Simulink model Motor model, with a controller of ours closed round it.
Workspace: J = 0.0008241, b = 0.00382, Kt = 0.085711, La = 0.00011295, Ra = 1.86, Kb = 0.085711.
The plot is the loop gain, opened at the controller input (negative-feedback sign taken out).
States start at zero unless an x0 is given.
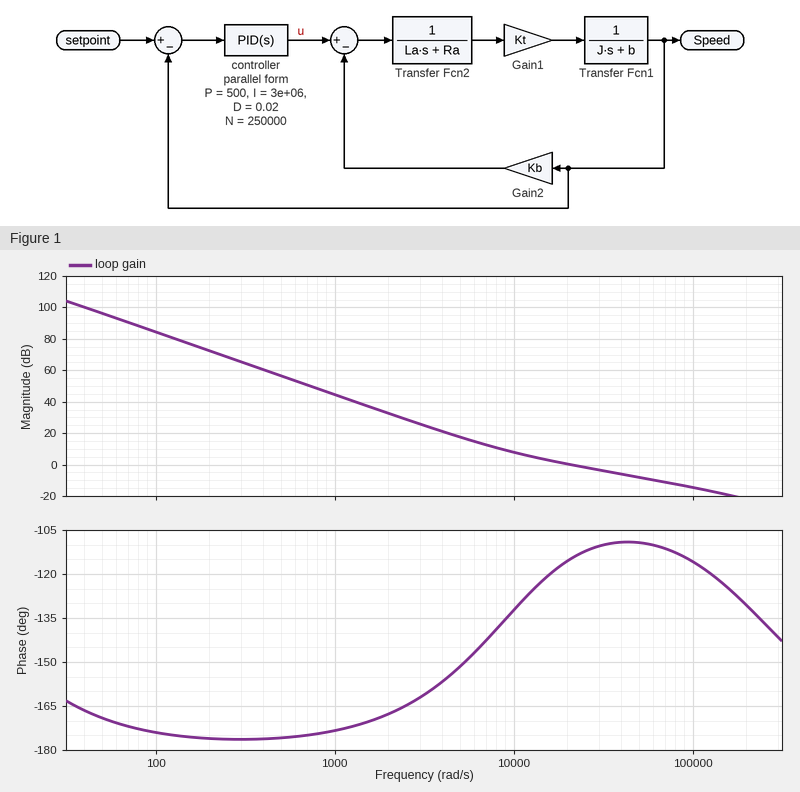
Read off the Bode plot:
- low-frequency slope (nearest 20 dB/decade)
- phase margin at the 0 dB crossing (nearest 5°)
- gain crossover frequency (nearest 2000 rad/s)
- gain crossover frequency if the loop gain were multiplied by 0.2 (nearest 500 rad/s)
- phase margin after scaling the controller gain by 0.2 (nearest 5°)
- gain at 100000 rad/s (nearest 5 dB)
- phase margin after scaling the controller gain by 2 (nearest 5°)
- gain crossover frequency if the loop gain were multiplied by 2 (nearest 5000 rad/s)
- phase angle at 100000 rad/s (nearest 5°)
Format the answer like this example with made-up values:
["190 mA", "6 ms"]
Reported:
["-40 dB/decade", "65°", "20000 rad/s", "6500 rad/s", "35°", "-15 dB", "70°", "40000 rad/s", "-115°"]
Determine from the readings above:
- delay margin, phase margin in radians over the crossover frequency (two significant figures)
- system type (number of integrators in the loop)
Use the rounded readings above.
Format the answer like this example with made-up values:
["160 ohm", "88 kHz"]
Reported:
["0.000057 s", "2"]
